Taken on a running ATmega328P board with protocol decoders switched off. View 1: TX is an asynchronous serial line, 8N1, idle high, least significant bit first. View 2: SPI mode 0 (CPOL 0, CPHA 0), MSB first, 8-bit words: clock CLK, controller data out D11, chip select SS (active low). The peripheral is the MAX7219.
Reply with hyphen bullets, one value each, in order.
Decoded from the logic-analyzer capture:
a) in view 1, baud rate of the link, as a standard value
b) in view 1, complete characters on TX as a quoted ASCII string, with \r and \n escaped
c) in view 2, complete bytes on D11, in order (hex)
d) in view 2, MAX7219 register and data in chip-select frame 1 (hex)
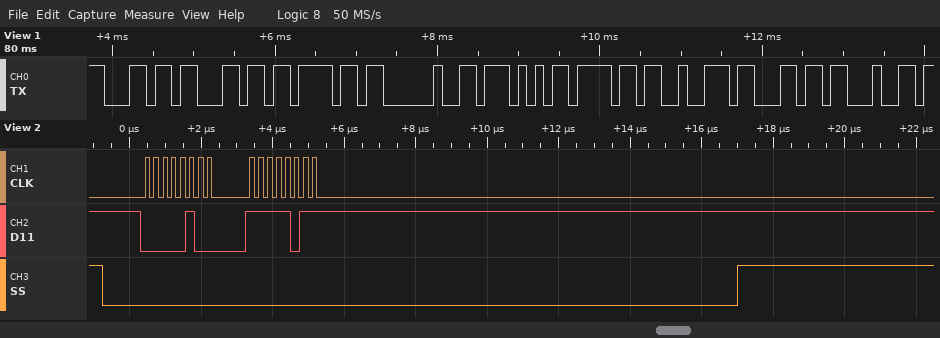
- 9600 baud
- "llo World"
- 0x04 0xFB
- register 0x4, data 0xFB
